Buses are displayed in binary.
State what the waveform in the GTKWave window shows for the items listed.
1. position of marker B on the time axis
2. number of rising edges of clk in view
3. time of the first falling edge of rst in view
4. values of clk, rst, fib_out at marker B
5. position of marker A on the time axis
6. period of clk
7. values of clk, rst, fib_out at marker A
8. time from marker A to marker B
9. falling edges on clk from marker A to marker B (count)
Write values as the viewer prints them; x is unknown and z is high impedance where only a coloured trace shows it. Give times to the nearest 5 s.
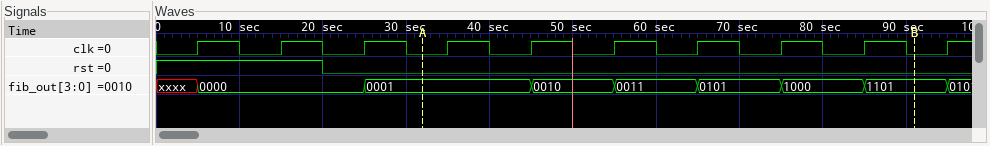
90 s
10
20 s
clk=0, rst=0, fib_out=1101
30 s
10 s
clk=0, rst=0, fib_out=0001
60 s
6
